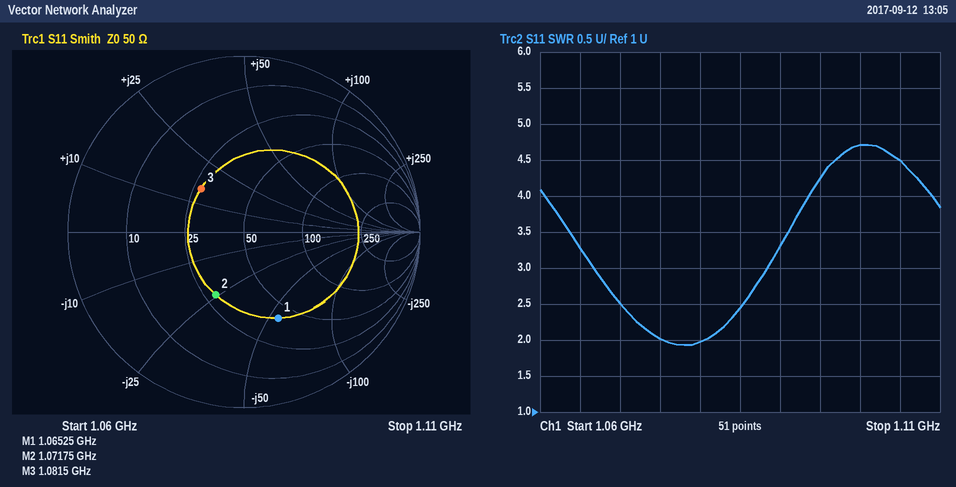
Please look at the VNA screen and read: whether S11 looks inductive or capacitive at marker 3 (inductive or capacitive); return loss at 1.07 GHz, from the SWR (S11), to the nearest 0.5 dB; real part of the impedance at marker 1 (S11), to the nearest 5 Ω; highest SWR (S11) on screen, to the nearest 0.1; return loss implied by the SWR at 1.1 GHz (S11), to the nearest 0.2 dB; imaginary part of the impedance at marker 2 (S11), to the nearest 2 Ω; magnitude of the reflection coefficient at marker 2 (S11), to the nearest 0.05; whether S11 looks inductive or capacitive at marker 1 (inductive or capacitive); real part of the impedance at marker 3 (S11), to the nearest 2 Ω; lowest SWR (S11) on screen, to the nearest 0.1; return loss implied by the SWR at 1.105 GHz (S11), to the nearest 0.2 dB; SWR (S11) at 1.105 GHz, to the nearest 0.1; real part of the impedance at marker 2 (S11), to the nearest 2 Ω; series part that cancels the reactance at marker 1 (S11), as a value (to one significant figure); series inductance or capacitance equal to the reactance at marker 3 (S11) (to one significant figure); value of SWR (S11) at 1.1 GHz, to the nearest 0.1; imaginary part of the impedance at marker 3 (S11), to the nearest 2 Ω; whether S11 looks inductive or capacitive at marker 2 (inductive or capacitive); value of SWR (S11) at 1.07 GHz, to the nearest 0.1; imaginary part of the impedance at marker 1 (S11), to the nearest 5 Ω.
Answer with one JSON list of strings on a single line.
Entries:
["inductive", "7.5 dB", "40 Ω", "4.7", "3.8 dB", "-24 Ω", "0.40", "capacitive", "28 Ω", "1.9", "4.0 dB", "4.5", "28 Ω", "8 nH", "2 nH", "4.7", "+16 Ω", "capacitive", "2.5", "-55 Ω"]
